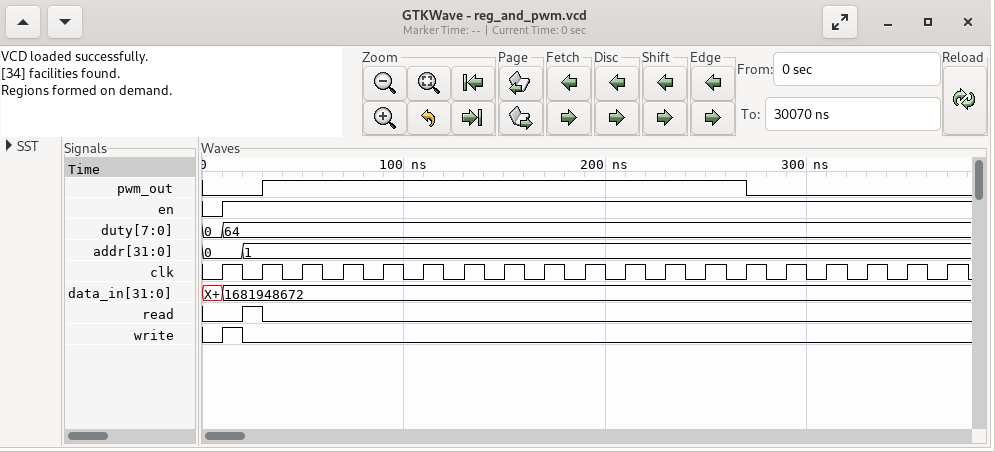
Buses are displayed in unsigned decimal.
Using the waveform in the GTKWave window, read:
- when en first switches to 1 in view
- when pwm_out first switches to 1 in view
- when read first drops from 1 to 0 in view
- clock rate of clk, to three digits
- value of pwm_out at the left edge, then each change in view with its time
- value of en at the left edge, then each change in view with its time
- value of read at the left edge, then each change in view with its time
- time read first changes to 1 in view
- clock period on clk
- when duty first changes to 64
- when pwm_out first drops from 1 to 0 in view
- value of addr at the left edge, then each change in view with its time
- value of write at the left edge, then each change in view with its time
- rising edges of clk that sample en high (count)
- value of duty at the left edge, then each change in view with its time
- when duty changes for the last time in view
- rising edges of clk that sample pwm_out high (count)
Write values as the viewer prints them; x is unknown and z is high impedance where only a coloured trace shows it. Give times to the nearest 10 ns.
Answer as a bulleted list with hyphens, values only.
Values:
- 10 ns
- 30 ns
- 30 ns
- 50.0 MHz
- 0, 1 at 30 ns, 0 at 270 ns
- 0, 1 at 10 ns
- 0, 1 at 20 ns, 0 at 30 ns
- 20 ns
- 20 ns
- 10 ns
- 270 ns
- 0, 1 at 20 ns
- 0, 1 at 10 ns, 0 at 20 ns
- 18
- 0, 64 at 10 ns
- 10 ns
- 12
